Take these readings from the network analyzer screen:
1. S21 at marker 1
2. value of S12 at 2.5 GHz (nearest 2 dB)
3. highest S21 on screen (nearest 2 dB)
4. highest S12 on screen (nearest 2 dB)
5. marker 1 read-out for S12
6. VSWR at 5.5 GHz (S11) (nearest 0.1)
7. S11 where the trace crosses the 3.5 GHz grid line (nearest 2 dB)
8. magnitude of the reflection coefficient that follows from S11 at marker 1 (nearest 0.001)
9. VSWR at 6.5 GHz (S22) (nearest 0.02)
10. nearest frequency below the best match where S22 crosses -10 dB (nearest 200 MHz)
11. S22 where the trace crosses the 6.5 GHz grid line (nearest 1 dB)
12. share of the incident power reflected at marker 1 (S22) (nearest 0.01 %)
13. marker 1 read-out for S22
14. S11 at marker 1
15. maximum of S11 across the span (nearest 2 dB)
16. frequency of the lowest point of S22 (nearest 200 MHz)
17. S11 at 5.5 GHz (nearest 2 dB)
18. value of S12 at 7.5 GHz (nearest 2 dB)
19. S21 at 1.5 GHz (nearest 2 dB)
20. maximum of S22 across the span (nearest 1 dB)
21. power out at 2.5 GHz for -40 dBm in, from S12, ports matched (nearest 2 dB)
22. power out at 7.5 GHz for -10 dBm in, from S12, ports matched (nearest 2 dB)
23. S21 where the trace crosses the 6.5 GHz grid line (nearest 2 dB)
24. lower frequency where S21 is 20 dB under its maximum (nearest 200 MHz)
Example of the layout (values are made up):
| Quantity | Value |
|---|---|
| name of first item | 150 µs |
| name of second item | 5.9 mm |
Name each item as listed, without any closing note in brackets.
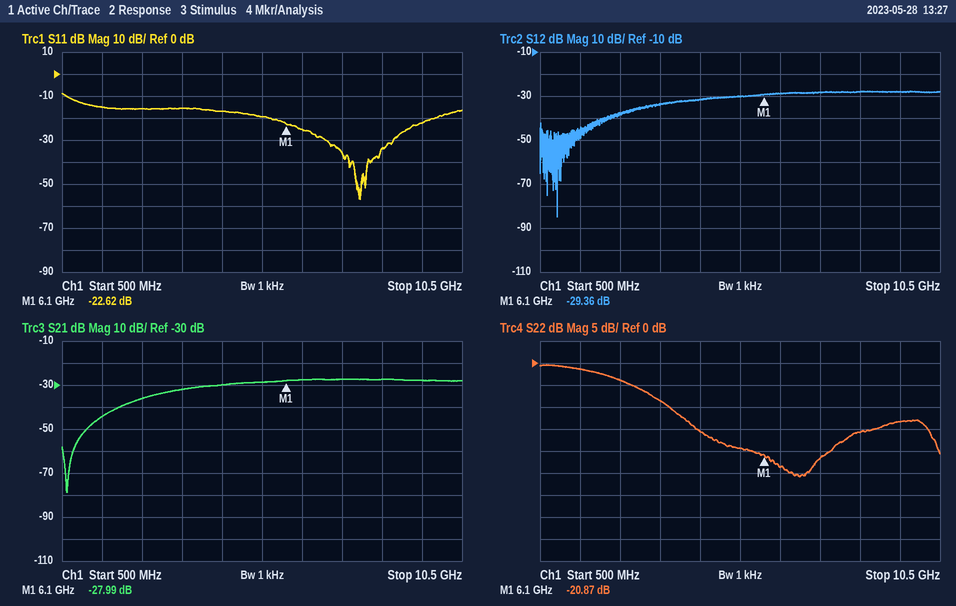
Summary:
| Quantity | Value |
|---|---|
| S21 at marker 1 | -27.99 dB |
| value of S12 at 2.5 GHz | -38 dB |
| highest S21 on screen | -28 dB |
| highest S12 on screen | -28 dB |
| marker 1 read-out for S12 | -29.36 dB |
| VSWR at 5.5 GHz (S11) | 1.2 |
| S11 where the trace crosses the 3.5 GHz grid line | -16 dB |
| magnitude of the reflection coefficient that follows from S11 at marker 1 | 0.074 |
| VSWR at 6.5 GHz (S22) | 1.14 |
| nearest frequency below the best match where S22 crosses -10 dB | 3.8 GHz |
| S22 where the trace crosses the 6.5 GHz grid line | -24 dB |
| share of the incident power reflected at marker 1 (S22) | 0.82 % |
| marker 1 read-out for S22 | -20.87 dB |
| S11 at marker 1 | -22.62 dB |
| maximum of S11 across the span | -8 dB |
| frequency of the lowest point of S22 | 7.0 GHz |
| S11 at 5.5 GHz | -20 dB |
| value of S12 at 7.5 GHz | -28 dB |
| S21 at 1.5 GHz | -44 dB |
| maximum of S22 across the span | 0 dB |
| power out at 2.5 GHz for -40 dBm in, from S12, ports matched | -78 dBm |
| power out at 7.5 GHz for -10 dBm in, from S12, ports matched | -38 dBm |
| S21 where the trace crosses the 6.5 GHz grid line | -28 dB |
| lower frequency where S21 is 20 dB under its maximum | 1.2 GHz |
